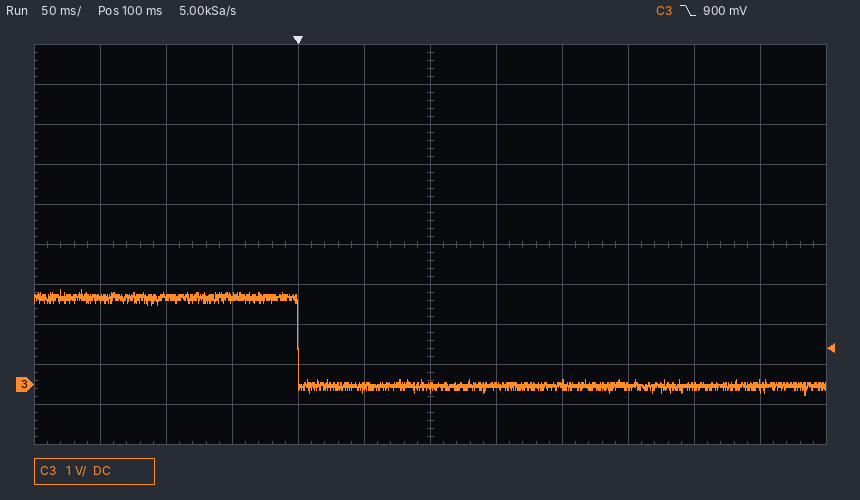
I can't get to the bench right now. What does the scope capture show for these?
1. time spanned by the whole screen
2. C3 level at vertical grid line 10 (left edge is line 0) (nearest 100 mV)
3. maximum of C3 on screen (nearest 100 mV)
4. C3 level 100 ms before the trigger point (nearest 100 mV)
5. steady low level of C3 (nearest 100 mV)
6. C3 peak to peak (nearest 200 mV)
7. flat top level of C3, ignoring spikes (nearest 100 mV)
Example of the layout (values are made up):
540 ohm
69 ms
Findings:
600 ms
0.0 V
2.4 V
2.2 V
0.0 V
2.6 V
2.2 V
